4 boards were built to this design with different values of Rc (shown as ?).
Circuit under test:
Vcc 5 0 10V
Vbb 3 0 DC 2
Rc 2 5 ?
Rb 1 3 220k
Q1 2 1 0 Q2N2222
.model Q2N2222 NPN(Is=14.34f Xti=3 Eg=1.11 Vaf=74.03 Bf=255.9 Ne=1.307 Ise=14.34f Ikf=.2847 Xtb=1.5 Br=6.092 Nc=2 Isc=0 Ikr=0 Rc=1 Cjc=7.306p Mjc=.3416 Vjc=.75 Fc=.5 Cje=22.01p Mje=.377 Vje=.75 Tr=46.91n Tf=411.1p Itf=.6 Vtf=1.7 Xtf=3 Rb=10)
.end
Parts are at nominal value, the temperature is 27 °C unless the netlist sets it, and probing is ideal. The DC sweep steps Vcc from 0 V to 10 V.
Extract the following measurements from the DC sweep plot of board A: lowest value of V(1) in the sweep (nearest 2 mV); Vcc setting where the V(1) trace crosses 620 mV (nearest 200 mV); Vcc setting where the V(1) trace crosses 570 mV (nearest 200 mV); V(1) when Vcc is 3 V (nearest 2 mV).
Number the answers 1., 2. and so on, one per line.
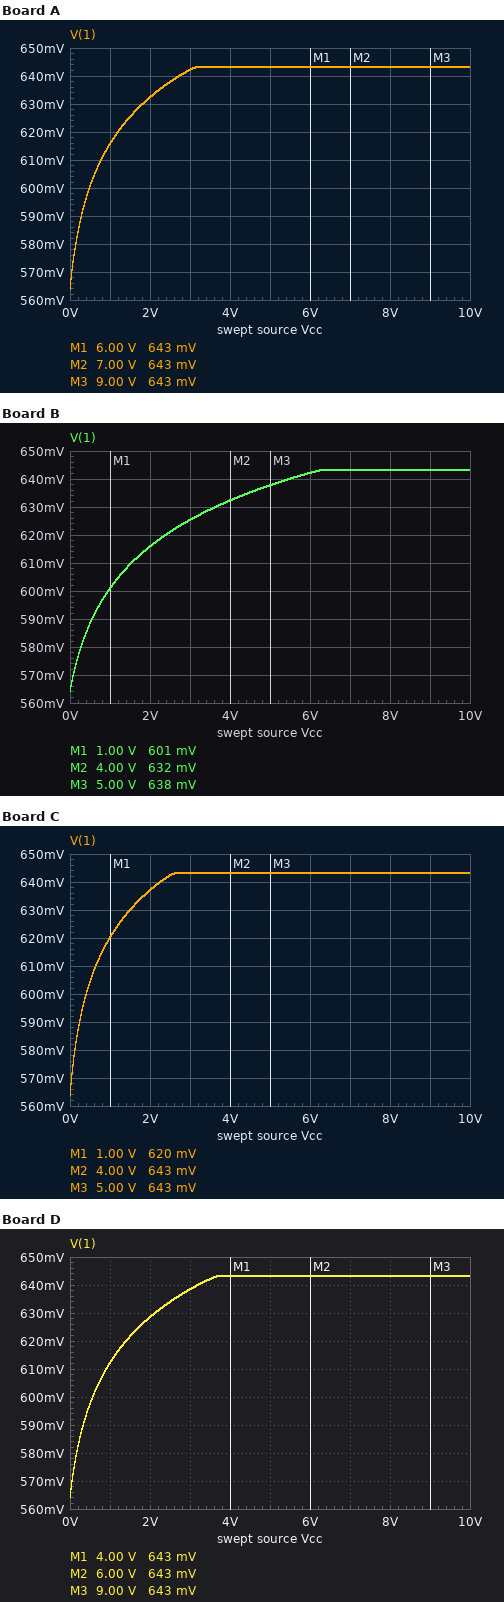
1. 564 mV
2. 1.2 V
3. 0 V
4. 642 mV
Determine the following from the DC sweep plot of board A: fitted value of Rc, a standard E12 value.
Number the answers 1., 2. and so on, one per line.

1. 3.3 kΩ
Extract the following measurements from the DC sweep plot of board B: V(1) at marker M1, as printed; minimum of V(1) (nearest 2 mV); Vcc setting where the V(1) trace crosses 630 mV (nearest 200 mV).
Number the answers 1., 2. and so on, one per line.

1. 601 mV
2. 564 mV
3. 3.6 V
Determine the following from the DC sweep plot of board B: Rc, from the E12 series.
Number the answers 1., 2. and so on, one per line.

1. 6.8 kΩ
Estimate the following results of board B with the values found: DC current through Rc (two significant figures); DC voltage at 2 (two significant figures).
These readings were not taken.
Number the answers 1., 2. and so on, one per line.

1. 940 µA
2. 3.6 V
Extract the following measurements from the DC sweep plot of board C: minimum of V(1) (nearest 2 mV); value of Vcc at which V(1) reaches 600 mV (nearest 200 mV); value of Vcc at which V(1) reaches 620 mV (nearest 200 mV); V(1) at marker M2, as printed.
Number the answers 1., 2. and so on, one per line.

1. 564 mV
2. 400 mV
3. 1.0 V
4. 643 mV
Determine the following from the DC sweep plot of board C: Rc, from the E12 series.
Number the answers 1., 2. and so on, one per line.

1. 2.7 kΩ
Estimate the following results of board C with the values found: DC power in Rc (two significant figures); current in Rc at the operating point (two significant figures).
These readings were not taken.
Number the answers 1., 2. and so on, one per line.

1. 2.6 mW
2. 980 µA
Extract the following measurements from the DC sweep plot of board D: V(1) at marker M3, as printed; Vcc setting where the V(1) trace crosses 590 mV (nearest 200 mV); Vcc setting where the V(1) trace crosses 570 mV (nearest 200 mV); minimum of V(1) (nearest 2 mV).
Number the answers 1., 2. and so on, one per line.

1. 643 mV
2. 400 mV
3. 0 V
4. 564 mV
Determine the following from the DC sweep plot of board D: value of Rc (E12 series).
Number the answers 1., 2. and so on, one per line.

1. 3.9 kΩ
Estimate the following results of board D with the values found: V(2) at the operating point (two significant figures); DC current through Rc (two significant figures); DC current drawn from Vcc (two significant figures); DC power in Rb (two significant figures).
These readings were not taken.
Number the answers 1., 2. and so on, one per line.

1. 6.2 V
2. 970 µA
3. 970 µA
4. 8.4 µW
